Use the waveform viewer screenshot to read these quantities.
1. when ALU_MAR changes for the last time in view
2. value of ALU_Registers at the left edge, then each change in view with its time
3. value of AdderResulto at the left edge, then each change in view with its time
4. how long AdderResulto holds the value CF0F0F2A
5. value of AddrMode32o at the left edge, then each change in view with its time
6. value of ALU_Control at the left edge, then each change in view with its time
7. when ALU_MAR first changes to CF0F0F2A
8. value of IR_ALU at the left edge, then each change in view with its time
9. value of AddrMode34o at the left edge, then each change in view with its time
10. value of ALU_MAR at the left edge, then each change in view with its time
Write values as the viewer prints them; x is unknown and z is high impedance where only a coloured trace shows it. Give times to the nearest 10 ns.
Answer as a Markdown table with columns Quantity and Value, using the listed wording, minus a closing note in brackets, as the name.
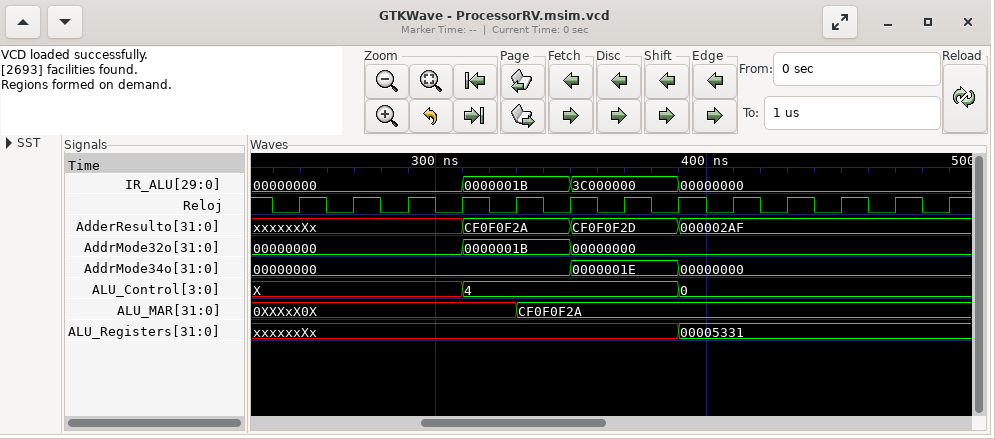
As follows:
| Quantity | Value |
|---|---|
| when ALU_MAR changes for the last time in view | 330 ns |
| value of ALU_Registers at the left edge, then each change in view with its time | xxxxxxXx, 00005331 at 390 ns |
| value of AdderResulto at the left edge, then each change in view with its time | xxxxxxXx, CF0F0F2A at 310 ns, CF0F0F2D at 350 ns, 000002AF at 390 ns |
| how long AdderResulto holds the value CF0F0F2A | 40 ns |
| value of AddrMode32o at the left edge, then each change in view with its time | 00000000, 0000001B at 310 ns, 00000000 at 350 ns |
| value of ALU_Control at the left edge, then each change in view with its time | X, 4 at 310 ns, 0 at 390 ns |
| when ALU_MAR first changes to CF0F0F2A | 330 ns |
| value of IR_ALU at the left edge, then each change in view with its time | 00000000, 0000001B at 310 ns, 3C000000 at 350 ns, 00000000 at 390 ns |
| value of AddrMode34o at the left edge, then each change in view with its time | 00000000, 0000001E at 350 ns, 00000000 at 390 ns |
| value of ALU_MAR at the left edge, then each change in view with its time | 0XXXxX0X, CF0F0F2A at 330 ns |
